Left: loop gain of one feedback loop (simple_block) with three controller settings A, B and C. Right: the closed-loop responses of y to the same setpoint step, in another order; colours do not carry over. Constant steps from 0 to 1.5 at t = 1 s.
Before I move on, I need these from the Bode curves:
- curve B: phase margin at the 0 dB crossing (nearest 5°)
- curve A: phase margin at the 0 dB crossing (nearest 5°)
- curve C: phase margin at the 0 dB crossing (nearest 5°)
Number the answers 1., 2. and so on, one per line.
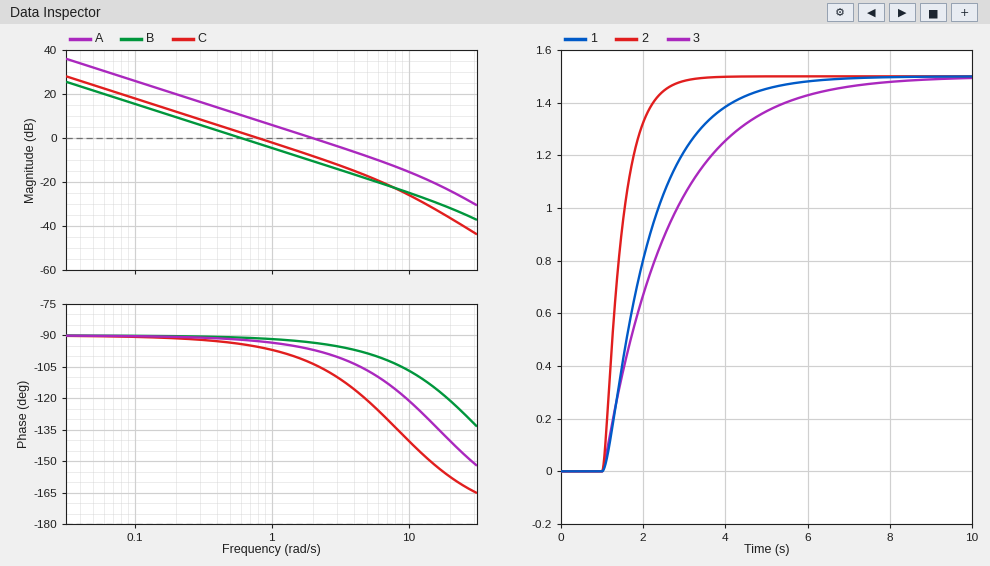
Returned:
1. 90°
2. 85°
3. 85°
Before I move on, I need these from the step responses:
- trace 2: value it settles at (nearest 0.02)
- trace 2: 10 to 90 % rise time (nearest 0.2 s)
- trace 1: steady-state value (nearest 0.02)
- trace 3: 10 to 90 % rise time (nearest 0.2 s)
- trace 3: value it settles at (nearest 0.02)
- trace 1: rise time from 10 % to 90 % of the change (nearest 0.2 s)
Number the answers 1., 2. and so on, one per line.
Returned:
1. 1.50
2. 1.0 s
3. 1.50
4. 3.6 s
5. 1.50
6. 2.4 s
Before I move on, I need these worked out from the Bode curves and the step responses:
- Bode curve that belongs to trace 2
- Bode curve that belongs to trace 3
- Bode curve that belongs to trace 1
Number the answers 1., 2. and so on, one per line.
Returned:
1. A
2. B
3. C
